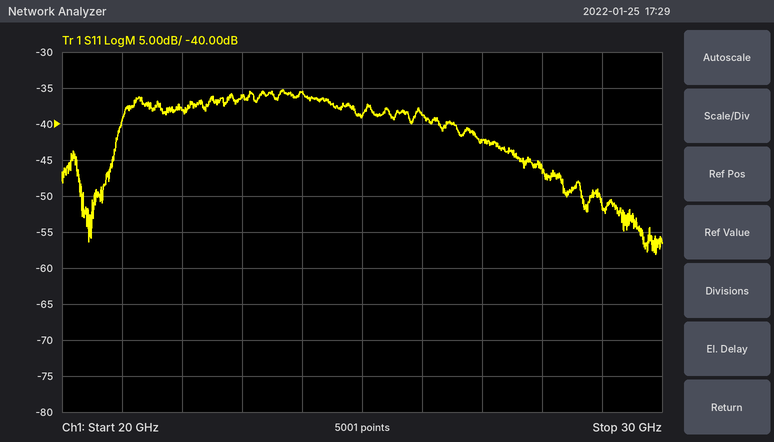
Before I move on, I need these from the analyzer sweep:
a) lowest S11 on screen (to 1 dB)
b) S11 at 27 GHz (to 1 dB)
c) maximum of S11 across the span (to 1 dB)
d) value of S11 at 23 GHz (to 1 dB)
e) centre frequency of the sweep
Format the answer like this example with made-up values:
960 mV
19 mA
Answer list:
-58 dB
-42 dB
-35 dB
-36 dB
25 GHz
